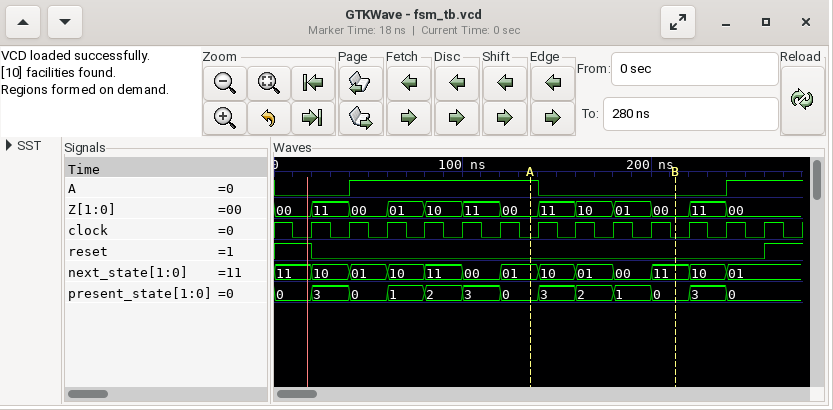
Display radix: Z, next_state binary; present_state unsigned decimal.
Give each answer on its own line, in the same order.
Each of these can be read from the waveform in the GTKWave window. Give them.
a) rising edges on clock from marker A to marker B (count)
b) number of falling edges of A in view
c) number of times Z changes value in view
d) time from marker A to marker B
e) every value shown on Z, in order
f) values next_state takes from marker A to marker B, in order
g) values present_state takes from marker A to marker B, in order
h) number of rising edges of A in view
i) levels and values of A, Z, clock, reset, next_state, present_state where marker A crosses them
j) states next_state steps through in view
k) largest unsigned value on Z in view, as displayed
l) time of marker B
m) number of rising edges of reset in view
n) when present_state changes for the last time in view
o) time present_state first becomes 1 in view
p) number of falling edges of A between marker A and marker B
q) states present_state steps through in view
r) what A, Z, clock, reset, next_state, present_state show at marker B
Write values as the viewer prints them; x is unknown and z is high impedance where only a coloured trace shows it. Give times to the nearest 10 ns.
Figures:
4
1
12
80 ns
00, 11, 00, 01, 10, 11, 00, 11, 10, 01, 00, 11, 00
01, 10, 01, 00, 11
0, 3, 2, 1, 0
2
A=1, Z=00, clock=0, reset=0, next_state=01, present_state=0
11, 10, 01, 10, 11, 00, 01, 10, 01, 00, 11, 10, 01
11
210 ns
1
240 ns
60 ns
1
0, 3, 0, 1, 2, 3, 0, 3, 2, 1, 0, 3, 0
A=0, Z=00, clock=0, reset=0, next_state=11, present_state=0
